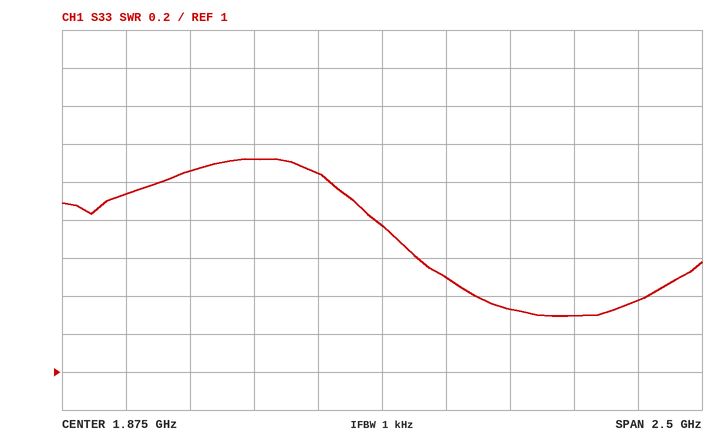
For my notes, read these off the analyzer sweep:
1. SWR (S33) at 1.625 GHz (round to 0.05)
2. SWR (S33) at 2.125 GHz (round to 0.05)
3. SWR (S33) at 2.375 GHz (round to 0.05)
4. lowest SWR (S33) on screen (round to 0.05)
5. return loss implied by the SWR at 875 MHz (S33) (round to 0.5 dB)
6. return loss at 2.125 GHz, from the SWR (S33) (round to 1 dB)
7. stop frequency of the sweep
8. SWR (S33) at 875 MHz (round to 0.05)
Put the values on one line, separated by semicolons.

2.05; 1.50; 1.35; 1.30; 10.0 dB; 14 dB; 3.125 GHz; 1.95
